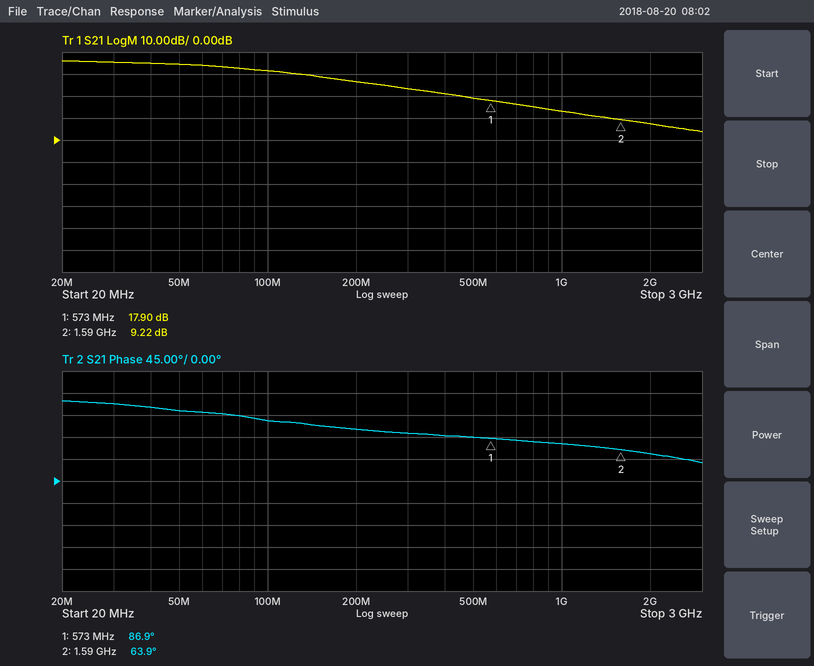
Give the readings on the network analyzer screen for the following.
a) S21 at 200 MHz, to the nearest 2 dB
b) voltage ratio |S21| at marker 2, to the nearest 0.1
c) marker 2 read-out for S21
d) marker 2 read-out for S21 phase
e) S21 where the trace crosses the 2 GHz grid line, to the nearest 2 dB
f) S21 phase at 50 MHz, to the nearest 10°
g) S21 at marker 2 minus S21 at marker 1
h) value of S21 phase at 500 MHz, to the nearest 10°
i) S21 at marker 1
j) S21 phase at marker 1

26 dB
2.9
9.22 dB
63.9°
8 dB
140°
-8.68 dB
90°
17.90 dB
86.9°
